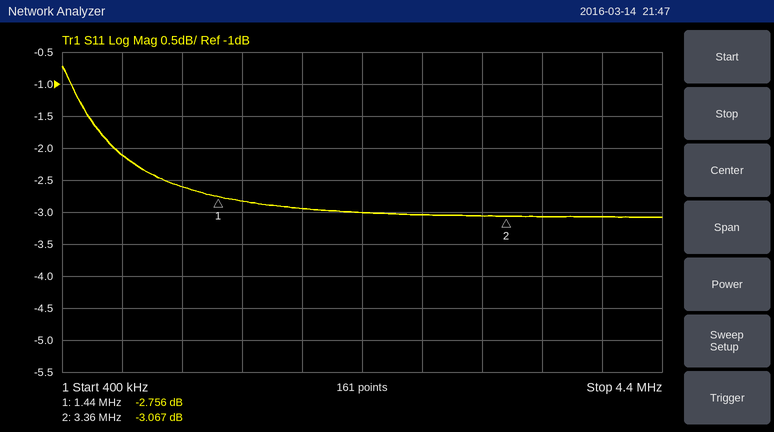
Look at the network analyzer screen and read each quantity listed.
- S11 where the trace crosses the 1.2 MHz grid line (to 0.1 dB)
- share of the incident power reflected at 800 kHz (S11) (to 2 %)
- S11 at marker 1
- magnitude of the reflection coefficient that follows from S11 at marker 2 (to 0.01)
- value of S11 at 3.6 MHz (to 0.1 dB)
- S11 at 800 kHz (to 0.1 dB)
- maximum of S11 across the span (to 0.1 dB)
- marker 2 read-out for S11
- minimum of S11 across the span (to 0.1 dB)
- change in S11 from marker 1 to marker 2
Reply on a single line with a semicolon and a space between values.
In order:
-2.6 dB; 62 %; -2.756 dB; 0.70; -3.1 dB; -2.1 dB; -0.7 dB; -3.067 dB; -3.1 dB; -0.311 dB
